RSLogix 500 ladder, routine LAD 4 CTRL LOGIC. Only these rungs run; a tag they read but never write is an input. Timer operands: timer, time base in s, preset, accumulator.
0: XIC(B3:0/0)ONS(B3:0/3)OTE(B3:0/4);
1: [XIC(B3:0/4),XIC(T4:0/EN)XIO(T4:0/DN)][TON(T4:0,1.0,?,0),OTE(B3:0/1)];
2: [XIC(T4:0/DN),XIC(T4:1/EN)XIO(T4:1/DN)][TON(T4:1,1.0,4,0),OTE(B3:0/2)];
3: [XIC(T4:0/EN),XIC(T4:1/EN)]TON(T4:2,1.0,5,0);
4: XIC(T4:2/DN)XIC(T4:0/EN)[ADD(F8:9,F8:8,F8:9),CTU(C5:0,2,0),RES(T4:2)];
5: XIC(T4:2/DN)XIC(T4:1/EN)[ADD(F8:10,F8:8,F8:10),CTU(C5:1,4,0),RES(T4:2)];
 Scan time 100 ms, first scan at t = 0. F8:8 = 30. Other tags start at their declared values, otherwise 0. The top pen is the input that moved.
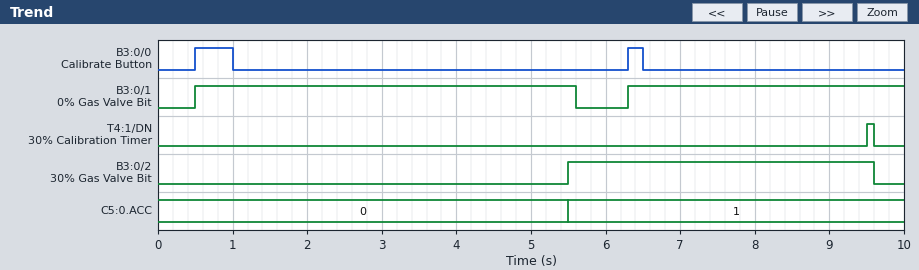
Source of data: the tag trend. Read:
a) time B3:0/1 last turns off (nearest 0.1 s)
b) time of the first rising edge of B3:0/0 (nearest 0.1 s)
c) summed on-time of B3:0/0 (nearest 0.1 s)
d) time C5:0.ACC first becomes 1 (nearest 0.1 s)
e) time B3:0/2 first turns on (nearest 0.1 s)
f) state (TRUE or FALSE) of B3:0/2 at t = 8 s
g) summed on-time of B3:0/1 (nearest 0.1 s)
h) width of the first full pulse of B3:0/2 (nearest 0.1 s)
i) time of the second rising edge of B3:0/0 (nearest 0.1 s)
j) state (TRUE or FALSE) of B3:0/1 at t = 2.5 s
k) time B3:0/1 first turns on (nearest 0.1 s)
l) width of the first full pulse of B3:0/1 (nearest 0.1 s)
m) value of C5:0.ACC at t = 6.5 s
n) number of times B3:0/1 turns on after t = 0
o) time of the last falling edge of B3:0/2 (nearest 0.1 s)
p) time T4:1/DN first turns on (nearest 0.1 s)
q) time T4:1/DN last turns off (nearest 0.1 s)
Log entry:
5.6 s
0.5 s
0.7 s
5.5 s
5.5 s
TRUE
8.8 s
4.1 s
6.3 s
TRUE
0.5 s
5.1 s
1
2
9.6 s
9.5 s
9.6 s
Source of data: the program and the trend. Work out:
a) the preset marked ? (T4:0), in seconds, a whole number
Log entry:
5 s
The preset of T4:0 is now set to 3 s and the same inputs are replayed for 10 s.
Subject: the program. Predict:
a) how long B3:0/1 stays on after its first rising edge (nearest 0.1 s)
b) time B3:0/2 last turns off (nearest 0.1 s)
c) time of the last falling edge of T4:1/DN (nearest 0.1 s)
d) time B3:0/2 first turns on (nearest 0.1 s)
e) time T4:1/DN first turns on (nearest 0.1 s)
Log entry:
3.1 s
7.6 s
7.6 s
3.5 s
7.5 s
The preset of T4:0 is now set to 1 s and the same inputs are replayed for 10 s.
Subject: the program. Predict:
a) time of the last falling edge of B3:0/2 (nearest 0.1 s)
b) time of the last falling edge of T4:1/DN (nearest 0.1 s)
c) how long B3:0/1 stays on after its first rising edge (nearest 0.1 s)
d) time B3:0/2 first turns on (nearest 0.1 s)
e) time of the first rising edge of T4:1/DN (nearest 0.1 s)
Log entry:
5.6 s
5.6 s
1.1 s
1.5 s
5.5 s
